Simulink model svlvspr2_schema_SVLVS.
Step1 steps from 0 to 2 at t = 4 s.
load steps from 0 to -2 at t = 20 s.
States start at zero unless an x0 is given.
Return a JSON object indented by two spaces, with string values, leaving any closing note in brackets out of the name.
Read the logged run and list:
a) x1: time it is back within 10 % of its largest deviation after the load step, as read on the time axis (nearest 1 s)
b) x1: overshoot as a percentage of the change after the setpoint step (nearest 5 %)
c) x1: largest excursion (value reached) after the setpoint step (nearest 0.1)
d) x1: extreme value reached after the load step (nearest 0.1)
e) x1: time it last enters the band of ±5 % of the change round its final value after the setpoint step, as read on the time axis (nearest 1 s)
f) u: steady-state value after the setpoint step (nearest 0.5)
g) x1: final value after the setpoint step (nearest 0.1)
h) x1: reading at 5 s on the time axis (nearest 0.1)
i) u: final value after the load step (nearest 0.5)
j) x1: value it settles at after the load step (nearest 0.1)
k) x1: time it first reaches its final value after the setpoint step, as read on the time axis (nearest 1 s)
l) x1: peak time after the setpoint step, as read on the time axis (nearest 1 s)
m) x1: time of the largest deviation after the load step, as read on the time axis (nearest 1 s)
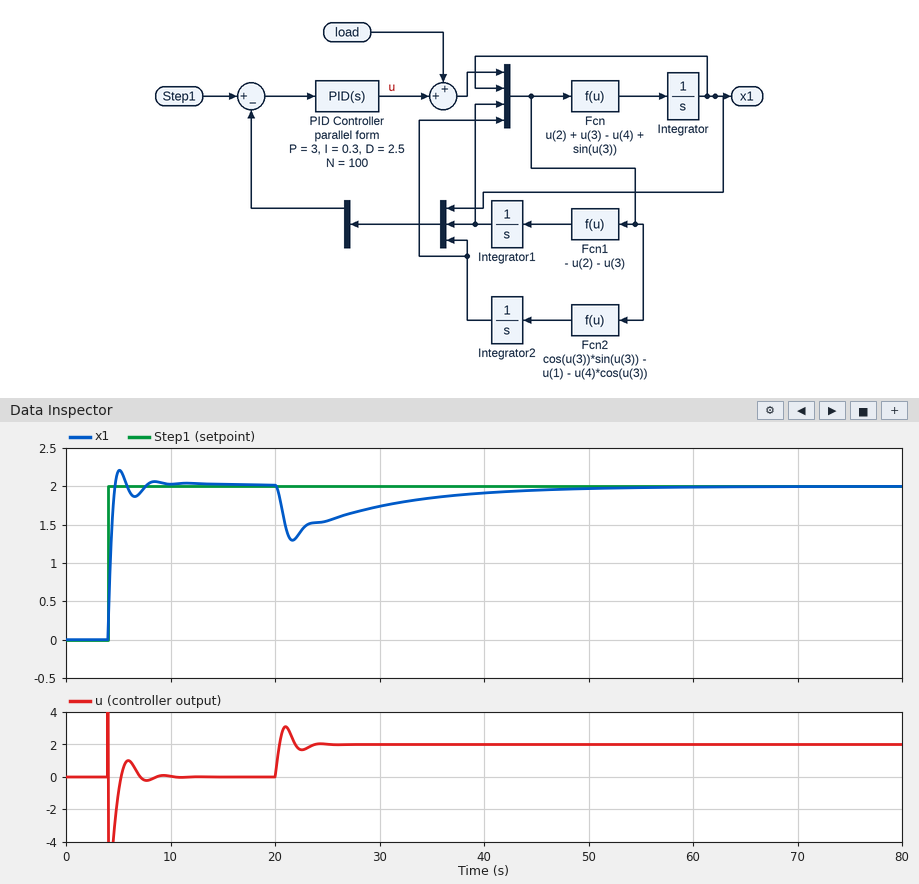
{
  "x1: time it is back within 10 % of its largest deviation after the load step, as read on the time axis": "42 s",
  "x1: overshoot as a percentage of the change after the setpoint step": "10 %",
  "x1: largest excursion (value reached) after the setpoint step": "2.2",
  "x1: extreme value reached after the load step": "1.3",
  "x1: time it last enters the band of ±5 % of the change round its final value after the setpoint step, as read on the time axis": "7 s",
  "u: steady-state value after the setpoint step": "0.0",
  "x1: final value after the setpoint step": "2.0",
  "x1: reading at 5 s on the time axis": "2.2",
  "u: final value after the load step": "2.0",
  "x1: value it settles at after the load step": "2.0",
  "x1: time it first reaches its final value after the setpoint step, as read on the time axis": "5 s",
  "x1: peak time after the setpoint step, as read on the time axis": "5 s",
  "x1: time of the largest deviation after the load step, as read on the time axis": "22 s"
}
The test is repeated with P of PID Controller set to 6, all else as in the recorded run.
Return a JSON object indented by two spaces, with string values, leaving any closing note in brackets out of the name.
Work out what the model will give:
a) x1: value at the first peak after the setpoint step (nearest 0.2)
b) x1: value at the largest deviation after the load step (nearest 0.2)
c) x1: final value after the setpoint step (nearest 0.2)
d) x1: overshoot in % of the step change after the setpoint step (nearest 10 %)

{
  "x1: value at the first peak after the setpoint step": "2.4",
  "x1: value at the largest deviation after the load step": "1.6",
  "x1: final value after the setpoint step": "2.0",
  "x1: overshoot in % of the step change after the setpoint step": "20 %"
}
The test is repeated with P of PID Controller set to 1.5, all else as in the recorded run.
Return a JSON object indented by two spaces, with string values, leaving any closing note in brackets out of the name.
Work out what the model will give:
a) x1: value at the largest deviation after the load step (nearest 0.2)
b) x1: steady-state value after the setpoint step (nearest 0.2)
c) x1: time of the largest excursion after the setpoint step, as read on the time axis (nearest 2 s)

{
  "x1: value at the largest deviation after the load step": "1.0",
  "x1: steady-state value after the setpoint step": "2.0",
  "x1: time of the largest excursion after the setpoint step, as read on the time axis": "10 s"
}
